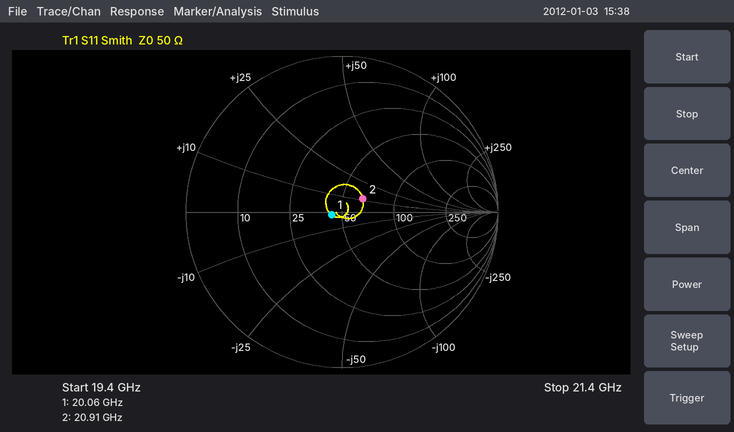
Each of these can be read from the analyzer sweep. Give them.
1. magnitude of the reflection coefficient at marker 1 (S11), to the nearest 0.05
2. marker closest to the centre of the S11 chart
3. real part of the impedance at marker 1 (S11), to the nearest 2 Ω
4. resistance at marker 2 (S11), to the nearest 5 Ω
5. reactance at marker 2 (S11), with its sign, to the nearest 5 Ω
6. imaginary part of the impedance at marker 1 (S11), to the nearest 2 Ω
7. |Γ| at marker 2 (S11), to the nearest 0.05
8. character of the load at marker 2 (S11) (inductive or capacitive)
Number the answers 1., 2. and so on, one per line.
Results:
1. 0.05
2. marker 1
3. 44 Ω
4. 65 Ω
5. +10 Ω
6. -2 Ω
7. 0.15
8. inductive
